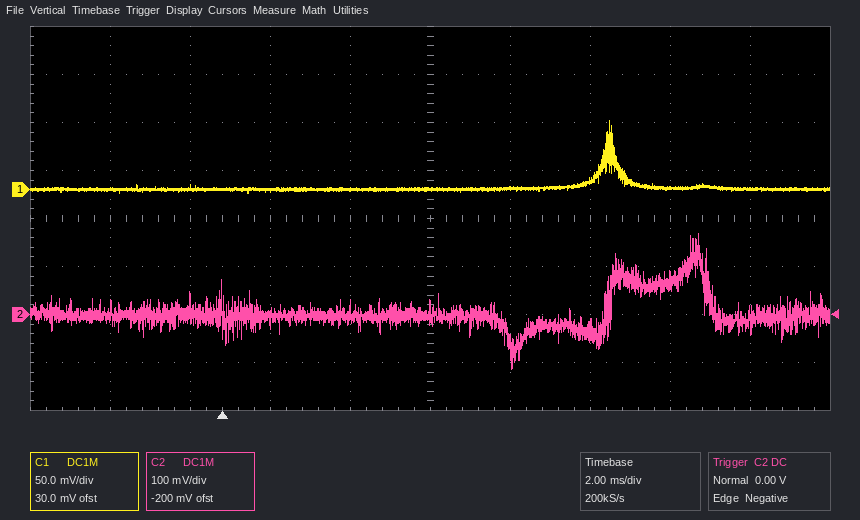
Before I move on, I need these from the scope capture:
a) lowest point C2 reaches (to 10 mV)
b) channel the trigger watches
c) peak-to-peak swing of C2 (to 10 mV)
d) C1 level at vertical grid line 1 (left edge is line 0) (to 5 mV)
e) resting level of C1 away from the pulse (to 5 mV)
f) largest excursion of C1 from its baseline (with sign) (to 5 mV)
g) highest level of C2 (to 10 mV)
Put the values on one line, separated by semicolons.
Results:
-110 mV; C2; 280 mV; 0 mV; 0 mV; +70 mV; 170 mV
